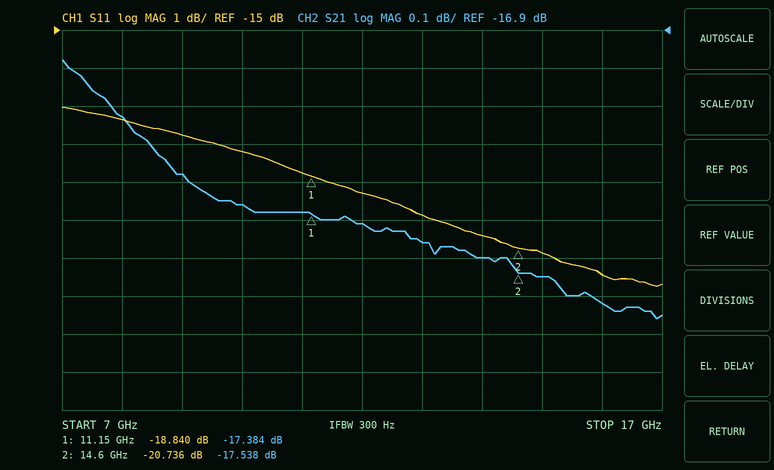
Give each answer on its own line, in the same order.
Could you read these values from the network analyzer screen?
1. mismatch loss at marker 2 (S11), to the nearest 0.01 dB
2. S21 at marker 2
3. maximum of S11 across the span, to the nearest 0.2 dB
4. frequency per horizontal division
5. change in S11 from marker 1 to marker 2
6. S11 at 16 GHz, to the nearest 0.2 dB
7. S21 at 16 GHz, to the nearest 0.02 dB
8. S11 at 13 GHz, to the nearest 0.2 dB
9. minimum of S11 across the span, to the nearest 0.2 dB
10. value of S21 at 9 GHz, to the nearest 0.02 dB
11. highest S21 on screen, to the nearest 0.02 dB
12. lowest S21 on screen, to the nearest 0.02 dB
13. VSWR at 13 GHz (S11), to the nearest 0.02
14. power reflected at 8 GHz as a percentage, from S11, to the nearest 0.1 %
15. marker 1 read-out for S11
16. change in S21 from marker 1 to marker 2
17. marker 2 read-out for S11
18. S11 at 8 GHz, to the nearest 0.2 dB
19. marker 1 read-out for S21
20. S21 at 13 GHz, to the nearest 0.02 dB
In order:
0.04 dB
-17.538 dB
-17.0 dB
1 GHz
-1.896 dB
-21.4 dB
-17.62 dB
-19.8 dB
-21.8 dB
-17.28 dB
-16.98 dB
-17.66 dB
1.22
1.8 %
-18.840 dB
-0.154 dB
-20.736 dB
-17.4 dB
-17.384 dB
-17.46 dB
